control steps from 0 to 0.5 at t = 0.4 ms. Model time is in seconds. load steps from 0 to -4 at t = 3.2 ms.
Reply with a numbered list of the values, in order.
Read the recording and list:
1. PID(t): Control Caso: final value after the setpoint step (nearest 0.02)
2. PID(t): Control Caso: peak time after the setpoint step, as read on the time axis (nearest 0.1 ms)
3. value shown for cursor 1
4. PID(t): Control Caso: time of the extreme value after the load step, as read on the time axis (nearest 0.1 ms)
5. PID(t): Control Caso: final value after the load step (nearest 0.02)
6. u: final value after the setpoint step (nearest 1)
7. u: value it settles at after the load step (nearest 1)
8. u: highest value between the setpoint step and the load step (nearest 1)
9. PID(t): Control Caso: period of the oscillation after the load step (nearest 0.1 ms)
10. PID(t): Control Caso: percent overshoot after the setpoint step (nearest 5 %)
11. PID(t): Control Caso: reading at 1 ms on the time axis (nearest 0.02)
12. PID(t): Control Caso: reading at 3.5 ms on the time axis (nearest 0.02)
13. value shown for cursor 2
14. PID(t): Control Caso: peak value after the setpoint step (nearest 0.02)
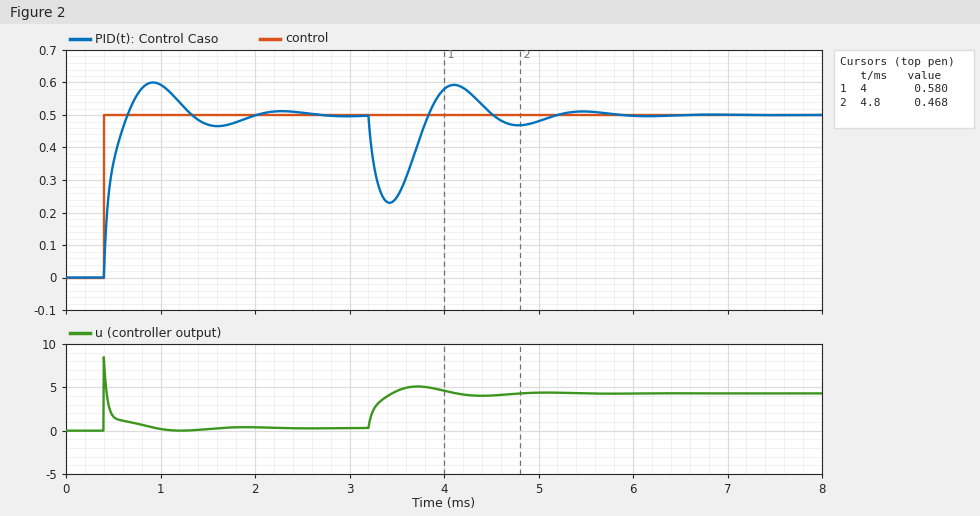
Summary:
1. 0.50
2. 0.9 ms
3. 0.580
4. 3.4 ms
5. 0.50
6. 0
7. 4
8. 8
9. 1.4 ms
10. 20 %
11. 0.60
12. 0.24
13. 0.468
14. 0.60
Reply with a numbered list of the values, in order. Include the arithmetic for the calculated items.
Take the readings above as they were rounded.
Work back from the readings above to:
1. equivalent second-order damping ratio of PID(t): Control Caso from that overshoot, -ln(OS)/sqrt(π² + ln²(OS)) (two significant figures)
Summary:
1. ln(0.2) = -1.609; 1.609 / sqrt(9.870 + 2.590) = 0.46
